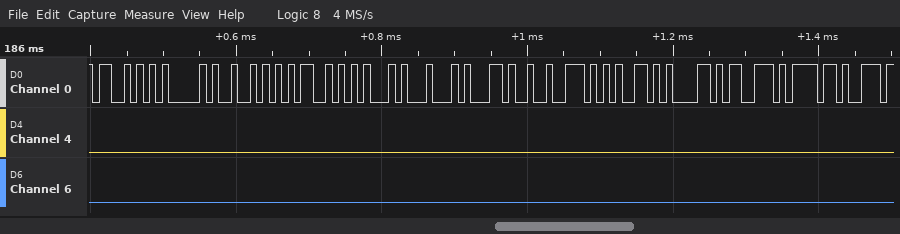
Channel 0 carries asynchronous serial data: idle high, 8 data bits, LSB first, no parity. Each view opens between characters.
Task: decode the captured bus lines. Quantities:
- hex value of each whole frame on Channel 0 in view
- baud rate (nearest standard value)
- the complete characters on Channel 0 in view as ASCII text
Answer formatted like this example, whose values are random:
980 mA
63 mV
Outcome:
53, 41, 52, 4D, 45, 44, 2C, 72, 65, 61, 73, 6F
115200 baud
"SARMED,reaso"
